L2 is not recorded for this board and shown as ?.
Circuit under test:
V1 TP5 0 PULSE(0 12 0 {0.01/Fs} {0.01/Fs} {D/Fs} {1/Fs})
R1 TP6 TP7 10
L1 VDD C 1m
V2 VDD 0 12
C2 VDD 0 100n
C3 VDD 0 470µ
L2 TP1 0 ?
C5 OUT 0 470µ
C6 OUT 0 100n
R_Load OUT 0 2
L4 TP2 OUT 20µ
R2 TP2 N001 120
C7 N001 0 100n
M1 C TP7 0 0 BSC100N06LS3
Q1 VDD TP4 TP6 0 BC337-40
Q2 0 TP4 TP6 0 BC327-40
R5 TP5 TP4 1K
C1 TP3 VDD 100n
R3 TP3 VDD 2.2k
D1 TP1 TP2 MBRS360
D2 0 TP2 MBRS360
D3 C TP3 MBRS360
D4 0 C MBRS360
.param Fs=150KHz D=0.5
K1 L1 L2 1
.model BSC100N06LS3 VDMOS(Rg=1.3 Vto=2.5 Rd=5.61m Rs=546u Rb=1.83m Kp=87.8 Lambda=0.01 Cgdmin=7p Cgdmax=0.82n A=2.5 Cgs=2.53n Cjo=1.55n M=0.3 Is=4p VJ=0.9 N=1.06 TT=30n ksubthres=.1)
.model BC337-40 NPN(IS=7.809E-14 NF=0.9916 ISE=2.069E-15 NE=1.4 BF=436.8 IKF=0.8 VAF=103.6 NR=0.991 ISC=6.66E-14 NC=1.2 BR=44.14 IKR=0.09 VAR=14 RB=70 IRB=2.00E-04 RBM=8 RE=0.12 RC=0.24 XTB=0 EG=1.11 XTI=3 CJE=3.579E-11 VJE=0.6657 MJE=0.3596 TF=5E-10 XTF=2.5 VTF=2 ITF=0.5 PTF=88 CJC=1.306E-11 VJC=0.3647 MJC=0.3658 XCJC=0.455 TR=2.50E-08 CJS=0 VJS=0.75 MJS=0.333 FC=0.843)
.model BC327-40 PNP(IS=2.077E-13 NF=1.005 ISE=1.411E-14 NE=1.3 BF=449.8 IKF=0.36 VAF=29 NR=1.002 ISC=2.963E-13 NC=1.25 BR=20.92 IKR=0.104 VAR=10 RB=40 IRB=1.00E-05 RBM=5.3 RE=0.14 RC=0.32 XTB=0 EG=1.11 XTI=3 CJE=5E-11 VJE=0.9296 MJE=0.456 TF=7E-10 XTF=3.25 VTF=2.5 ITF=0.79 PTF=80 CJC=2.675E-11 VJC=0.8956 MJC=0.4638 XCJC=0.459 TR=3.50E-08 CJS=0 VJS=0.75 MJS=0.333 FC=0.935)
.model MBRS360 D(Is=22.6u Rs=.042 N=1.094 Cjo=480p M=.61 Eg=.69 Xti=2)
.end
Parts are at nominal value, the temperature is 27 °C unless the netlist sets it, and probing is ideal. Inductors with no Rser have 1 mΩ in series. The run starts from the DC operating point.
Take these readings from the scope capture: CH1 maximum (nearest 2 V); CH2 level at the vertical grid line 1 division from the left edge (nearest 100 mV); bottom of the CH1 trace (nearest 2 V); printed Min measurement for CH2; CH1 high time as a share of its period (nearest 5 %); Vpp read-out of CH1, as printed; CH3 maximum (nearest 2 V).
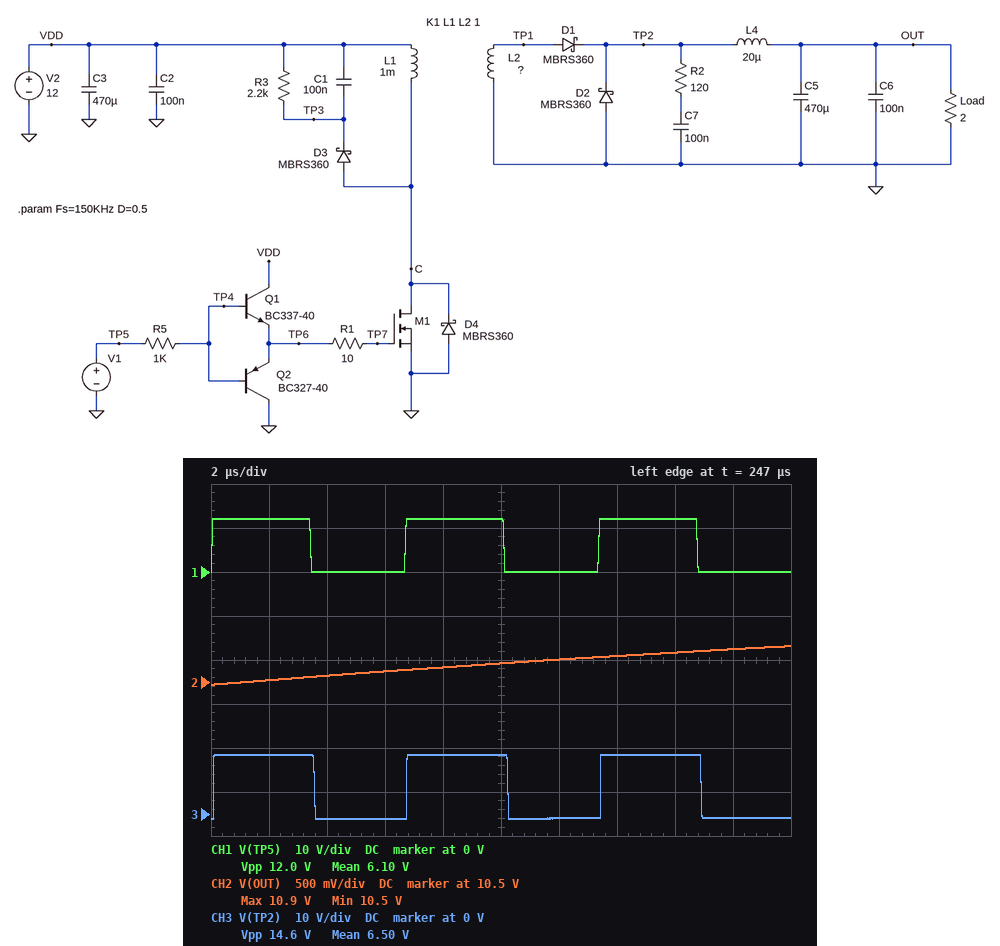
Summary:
12 V
10.5 V
0 V
10.5 V
50 %
12.0 V
14 V
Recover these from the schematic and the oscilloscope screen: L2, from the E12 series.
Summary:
1.5 mH
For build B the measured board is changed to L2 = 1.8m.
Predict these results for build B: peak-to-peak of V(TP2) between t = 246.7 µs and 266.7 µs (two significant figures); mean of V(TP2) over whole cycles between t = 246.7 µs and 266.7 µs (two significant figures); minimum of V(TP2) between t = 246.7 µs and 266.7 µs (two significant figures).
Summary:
16 V
7.2 V
-1.2 V
